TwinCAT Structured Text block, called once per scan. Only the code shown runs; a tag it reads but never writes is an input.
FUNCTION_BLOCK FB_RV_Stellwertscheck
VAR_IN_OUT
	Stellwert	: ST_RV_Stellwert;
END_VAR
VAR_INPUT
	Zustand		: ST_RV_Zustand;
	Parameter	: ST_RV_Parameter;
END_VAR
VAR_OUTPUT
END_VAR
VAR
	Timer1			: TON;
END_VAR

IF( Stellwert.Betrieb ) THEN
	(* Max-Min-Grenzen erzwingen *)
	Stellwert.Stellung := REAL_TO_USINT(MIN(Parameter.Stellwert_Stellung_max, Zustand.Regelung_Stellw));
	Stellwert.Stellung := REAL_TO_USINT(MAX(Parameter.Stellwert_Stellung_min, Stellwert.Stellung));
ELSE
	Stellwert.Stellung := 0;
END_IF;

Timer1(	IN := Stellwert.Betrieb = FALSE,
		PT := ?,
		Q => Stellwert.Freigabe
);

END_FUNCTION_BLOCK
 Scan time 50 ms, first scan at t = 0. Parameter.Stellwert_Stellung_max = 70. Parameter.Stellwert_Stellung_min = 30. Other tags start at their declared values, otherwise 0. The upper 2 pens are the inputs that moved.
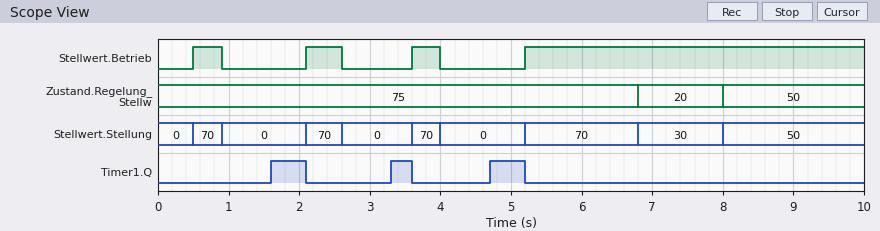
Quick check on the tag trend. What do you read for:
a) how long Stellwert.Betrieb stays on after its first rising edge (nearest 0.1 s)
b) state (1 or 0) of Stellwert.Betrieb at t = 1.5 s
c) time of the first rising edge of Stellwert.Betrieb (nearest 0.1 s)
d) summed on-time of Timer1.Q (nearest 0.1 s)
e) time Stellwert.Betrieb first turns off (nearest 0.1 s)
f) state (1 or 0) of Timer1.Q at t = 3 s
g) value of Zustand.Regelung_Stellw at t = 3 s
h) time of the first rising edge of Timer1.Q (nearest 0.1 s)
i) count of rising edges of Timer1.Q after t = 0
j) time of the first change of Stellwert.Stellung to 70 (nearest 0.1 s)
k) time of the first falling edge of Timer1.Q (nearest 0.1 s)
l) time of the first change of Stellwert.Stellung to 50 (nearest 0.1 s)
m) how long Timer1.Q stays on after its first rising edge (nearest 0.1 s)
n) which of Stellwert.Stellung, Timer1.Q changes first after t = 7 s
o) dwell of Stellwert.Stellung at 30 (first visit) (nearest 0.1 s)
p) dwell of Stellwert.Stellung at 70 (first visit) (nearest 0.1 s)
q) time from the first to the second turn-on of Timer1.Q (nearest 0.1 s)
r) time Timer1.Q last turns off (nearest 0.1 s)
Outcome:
0.4 s
0
0.5 s
1.3 s
0.9 s
0
75
1.6 s
3
0.5 s
2.1 s
8.0 s
0.5 s
Stellwert.Stellung
1.2 s
0.4 s
1.7 s
5.2 s
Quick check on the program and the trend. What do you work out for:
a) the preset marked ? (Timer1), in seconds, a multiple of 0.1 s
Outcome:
0.7 s
